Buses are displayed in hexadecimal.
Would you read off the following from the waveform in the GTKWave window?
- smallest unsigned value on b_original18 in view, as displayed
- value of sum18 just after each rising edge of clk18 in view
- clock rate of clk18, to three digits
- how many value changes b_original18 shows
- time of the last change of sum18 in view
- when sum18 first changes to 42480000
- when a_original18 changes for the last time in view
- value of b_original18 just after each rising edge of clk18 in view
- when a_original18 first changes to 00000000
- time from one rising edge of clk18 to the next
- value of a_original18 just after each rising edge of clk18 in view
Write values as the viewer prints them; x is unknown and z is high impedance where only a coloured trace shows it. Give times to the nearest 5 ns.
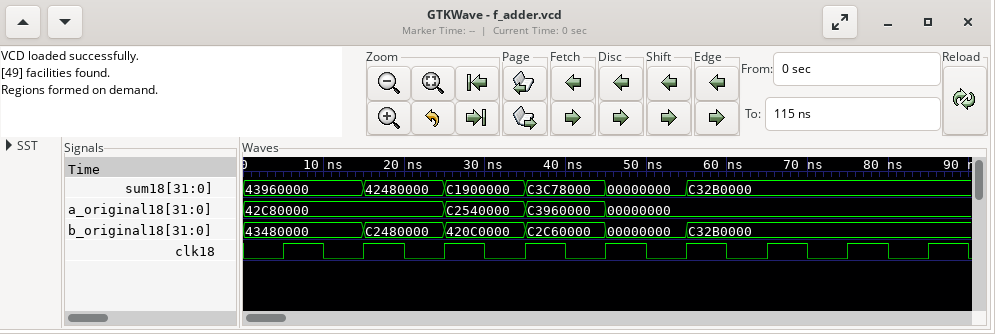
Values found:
00000000
43960000, 42480000, C1900000, C3C78000, 00000000, C32B0000, C32B0000, C32B0000, C32B0000
100 MHz
5
55 ns
15 ns
45 ns
43480000, C2480000, 420C0000, C2C60000, 00000000, C32B0000, C32B0000, C32B0000, C32B0000
45 ns
10 ns
42C80000, 42C80000, C2540000, C3960000, 00000000, 00000000, 00000000, 00000000, 00000000
